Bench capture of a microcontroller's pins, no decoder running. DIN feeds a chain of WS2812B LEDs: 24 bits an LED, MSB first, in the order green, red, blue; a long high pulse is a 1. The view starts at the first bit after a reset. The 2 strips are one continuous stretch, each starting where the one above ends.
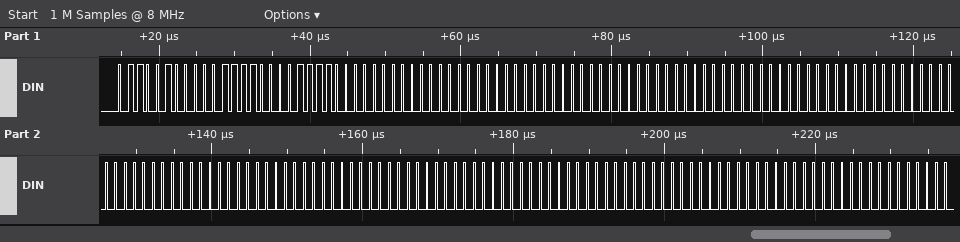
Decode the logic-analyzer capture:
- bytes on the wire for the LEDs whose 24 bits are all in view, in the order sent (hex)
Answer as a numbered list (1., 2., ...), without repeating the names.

1. 64 1E 1E 00 00 00 00 00 00 00 00 00 00 00 00 00 00 00 00 00 00
